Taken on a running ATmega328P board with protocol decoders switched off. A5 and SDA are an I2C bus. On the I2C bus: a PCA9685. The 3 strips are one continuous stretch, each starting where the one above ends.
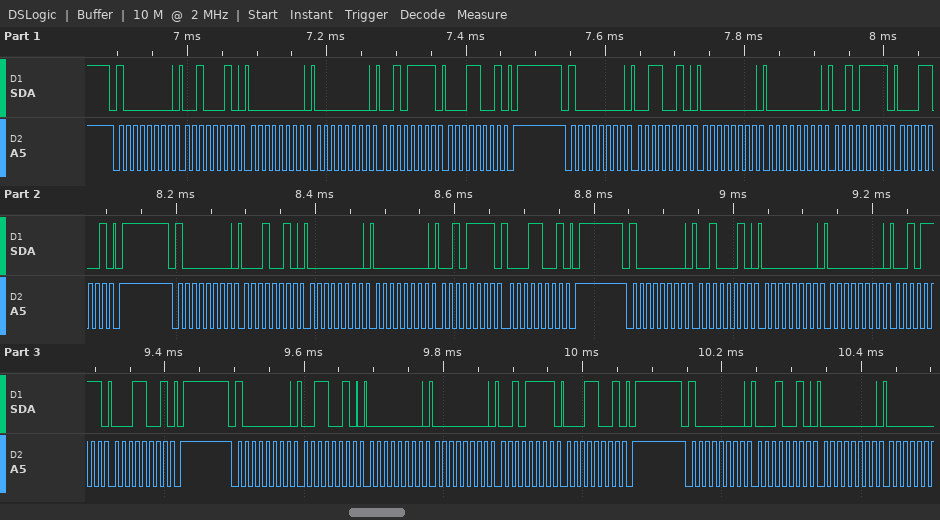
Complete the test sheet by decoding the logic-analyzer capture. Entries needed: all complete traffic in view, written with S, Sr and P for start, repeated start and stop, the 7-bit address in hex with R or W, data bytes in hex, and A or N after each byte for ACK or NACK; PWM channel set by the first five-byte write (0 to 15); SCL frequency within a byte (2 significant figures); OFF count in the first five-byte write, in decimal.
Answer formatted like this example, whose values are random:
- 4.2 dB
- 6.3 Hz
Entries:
- S 40W A 22 A 00 A 00 A 2F A 19 A P S 40W A 32 A 00 A 00 A 2F A 19 A P S 40W A 12 A 00 A 00 A 2F A 19 A P S 40W A 22 A 00 A 00 A 2F A 19 A P S 40W A 32 A 00 A 00 A 2F A 19 A P S 40W A 12 A 00 A
- 7
- 100 kHz
- 6447
